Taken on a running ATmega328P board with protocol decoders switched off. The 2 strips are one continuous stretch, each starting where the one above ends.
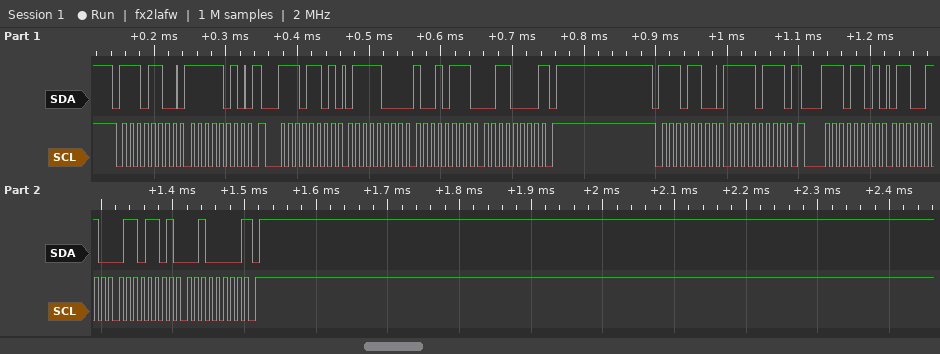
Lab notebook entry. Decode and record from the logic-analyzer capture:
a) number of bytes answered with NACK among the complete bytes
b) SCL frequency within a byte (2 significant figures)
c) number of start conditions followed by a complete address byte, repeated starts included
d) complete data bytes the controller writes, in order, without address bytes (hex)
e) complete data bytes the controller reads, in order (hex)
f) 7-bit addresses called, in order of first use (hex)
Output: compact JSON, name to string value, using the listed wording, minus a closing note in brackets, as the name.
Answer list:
{"number of bytes answered with NACK among the complete bytes": "2", "SCL frequency within a byte": "100 kHz", "number of start conditions followed by a complete address byte, repeated starts included": "4", "complete data bytes the controller writes, in order, without address bytes": "FA F7", "complete data bytes the controller reads, in order": "78 97 30 66 6D 20", "7-bit addresses called, in order of first use": "0x76"}
